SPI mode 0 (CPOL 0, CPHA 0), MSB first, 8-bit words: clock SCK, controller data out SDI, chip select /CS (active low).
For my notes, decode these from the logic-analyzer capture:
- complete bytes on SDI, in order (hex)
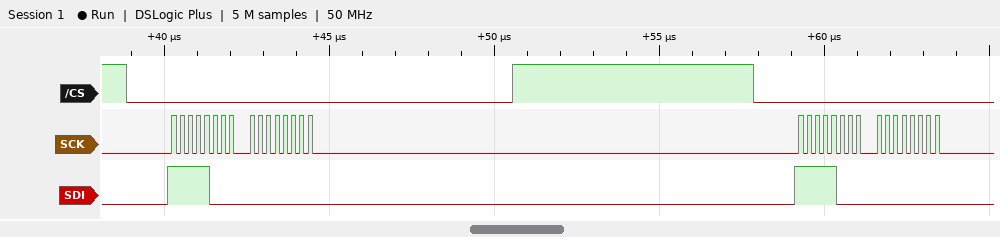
0xF8 0x00 0xF8 0x00
